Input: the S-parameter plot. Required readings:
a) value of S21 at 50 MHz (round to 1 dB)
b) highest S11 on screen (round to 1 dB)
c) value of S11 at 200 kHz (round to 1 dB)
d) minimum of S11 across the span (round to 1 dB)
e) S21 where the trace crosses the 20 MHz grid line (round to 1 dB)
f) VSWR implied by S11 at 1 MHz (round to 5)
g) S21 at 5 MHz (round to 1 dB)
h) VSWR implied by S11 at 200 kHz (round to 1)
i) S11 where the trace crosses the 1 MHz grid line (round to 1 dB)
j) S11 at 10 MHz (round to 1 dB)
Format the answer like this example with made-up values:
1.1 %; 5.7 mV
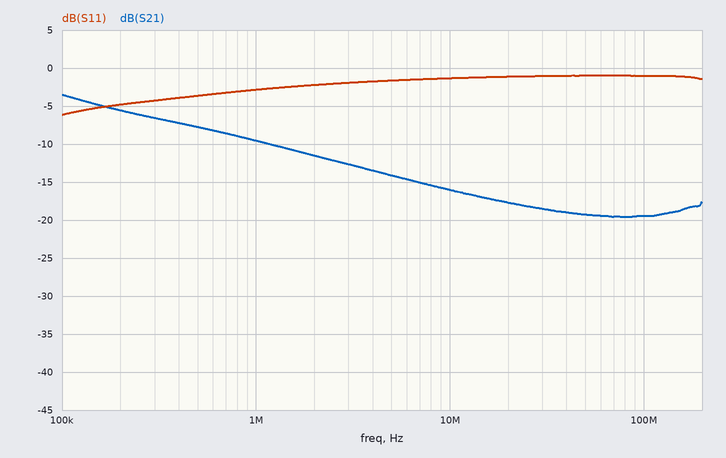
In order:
-19 dB; -1 dB; -5 dB; -6 dB; -18 dB; 5; -14 dB; 4; -3 dB; -1 dB
